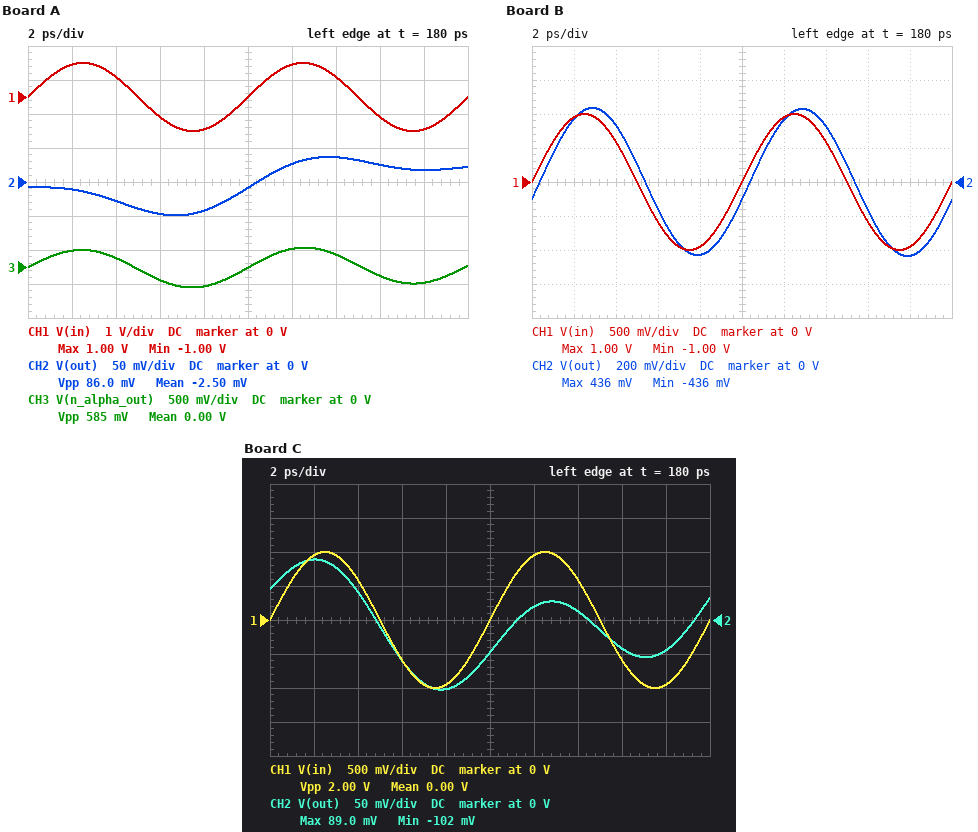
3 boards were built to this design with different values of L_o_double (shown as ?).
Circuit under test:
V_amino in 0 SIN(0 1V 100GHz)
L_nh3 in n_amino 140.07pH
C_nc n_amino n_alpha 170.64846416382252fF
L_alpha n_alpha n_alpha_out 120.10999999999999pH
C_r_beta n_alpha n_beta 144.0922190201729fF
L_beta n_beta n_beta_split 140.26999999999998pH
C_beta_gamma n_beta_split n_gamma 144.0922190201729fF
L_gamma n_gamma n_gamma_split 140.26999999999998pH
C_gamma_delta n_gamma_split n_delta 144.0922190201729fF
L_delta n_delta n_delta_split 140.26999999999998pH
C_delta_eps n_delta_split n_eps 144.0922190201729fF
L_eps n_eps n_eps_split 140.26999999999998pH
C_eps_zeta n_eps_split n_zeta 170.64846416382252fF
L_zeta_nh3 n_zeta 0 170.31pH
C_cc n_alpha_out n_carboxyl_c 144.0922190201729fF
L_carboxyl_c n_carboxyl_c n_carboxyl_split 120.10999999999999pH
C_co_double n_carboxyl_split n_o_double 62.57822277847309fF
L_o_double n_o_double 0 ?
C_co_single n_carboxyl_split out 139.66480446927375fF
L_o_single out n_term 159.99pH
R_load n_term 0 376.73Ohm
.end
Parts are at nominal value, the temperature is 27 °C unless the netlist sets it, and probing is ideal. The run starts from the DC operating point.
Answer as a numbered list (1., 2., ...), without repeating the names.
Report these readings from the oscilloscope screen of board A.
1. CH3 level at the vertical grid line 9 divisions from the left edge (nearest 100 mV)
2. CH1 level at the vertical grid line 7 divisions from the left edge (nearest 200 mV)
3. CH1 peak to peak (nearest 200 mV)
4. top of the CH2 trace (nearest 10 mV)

1. -200 mV
2. 600 mV
3. 2.0 V
4. 40 mV
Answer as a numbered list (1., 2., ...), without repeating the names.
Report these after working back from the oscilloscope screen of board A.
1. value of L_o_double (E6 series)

1. 47 pH
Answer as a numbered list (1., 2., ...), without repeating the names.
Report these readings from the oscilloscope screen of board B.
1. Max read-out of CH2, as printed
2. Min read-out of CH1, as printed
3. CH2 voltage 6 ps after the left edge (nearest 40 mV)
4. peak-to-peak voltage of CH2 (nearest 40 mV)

1. 436 mV
2. -1.00 V
3. -160 mV
4. 880 mV
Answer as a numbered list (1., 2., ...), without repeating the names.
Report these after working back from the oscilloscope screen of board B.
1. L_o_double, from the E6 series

1. 470 pH
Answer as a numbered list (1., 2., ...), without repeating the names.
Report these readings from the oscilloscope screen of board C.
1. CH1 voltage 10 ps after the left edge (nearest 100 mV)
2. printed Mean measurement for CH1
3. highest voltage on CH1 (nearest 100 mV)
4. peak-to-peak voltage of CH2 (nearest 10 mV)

1. 0 V
2. 0.00 V
3. 1.0 V
4. 190 mV
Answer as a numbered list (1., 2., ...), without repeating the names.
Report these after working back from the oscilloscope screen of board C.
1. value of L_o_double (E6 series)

1. 68 pH
